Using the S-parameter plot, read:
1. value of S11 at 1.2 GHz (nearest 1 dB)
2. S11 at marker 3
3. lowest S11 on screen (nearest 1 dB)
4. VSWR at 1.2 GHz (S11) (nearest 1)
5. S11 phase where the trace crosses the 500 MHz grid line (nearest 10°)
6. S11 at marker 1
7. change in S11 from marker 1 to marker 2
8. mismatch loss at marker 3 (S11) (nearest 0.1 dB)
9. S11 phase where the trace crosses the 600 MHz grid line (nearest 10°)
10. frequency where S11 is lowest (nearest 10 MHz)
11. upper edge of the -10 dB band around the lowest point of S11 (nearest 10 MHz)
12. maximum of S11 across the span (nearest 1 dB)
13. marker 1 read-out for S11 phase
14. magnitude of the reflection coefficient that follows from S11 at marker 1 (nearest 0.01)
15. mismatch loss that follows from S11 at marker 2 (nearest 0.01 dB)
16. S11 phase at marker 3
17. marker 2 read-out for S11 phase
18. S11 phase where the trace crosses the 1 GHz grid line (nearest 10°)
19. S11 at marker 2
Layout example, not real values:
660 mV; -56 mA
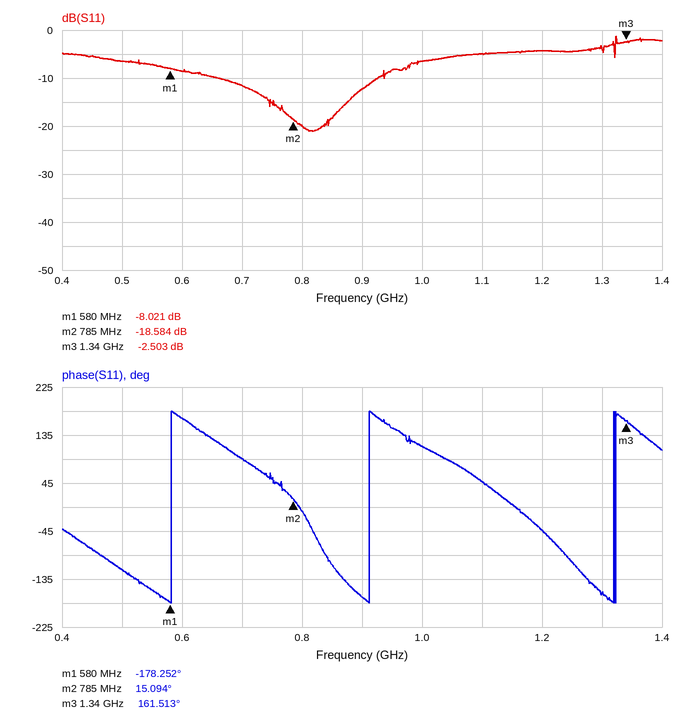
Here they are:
-4 dB; -2.503 dB; -21 dB; 4; -120°; -8.021 dB; -10.563 dB; 3.6 dB; 170°; 810 MHz; 930 MHz; -1 dB; -178.252°; 0.40; 0.06 dB; 161.513°; 15.094°; 110°; -18.584 dB
